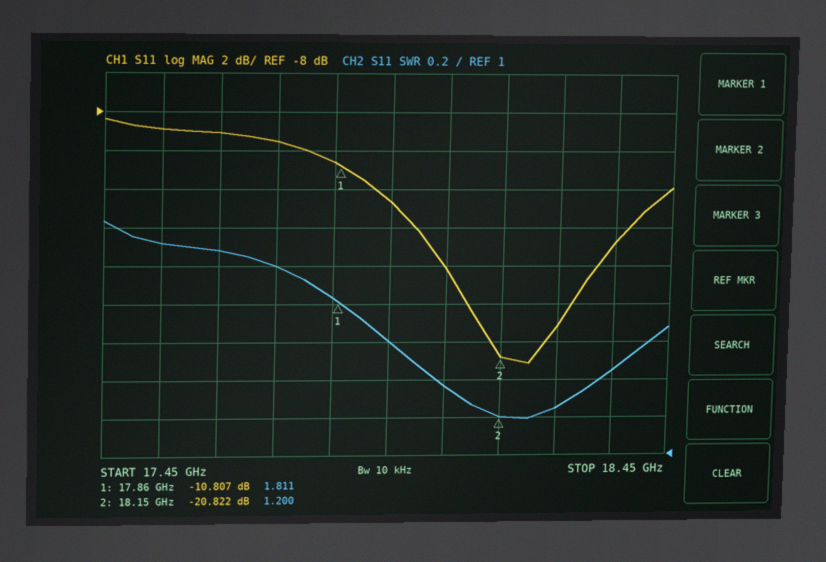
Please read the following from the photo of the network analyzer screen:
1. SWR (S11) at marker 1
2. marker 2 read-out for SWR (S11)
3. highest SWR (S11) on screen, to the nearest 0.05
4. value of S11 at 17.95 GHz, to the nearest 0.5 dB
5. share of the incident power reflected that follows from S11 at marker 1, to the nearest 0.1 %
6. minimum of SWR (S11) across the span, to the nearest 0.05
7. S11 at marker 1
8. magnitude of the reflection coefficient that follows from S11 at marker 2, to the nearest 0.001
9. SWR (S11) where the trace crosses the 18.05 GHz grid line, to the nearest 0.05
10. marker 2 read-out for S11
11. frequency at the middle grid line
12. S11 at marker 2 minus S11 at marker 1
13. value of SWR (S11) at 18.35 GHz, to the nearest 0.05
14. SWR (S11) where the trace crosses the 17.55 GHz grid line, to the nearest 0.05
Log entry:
1.811
1.200
2.25
-12.5 dB
8.3 %
1.20
-10.807 dB
0.091
1.35
-20.822 dB
17.95 GHz
-10.015 dB
1.45
2.10
